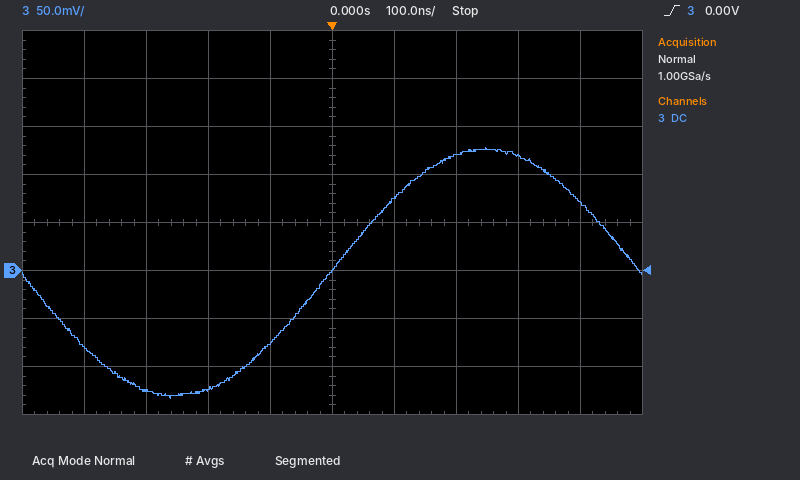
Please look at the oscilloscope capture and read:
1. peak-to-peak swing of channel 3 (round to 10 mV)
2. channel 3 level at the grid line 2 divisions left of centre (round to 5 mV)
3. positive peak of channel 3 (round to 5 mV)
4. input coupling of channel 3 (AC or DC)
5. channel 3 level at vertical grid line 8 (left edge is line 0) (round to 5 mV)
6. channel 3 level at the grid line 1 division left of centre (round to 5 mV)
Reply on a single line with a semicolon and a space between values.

260 mV; -125 mV; 130 mV; DC; 120 mV; -75 mV
